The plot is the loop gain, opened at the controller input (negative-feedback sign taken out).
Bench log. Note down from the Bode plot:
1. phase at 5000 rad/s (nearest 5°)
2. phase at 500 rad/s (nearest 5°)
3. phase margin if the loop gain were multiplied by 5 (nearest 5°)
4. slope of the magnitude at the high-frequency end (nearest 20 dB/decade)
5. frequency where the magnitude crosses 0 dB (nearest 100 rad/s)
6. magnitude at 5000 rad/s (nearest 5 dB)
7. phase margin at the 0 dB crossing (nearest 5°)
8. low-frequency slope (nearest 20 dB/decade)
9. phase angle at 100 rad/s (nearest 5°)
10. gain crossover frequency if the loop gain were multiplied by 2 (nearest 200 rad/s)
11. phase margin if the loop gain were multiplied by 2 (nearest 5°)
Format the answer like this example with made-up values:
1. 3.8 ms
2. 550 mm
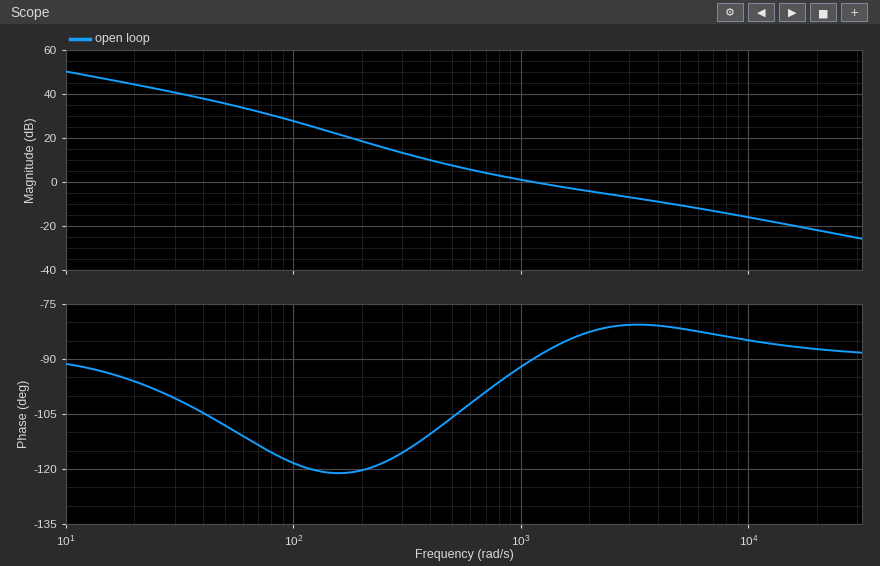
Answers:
1. -80°
2. -105°
3. 95°
4. -20 dB/decade
5. 1100 rad/s
6. -10 dB
7. 90°
8. -20 dB/decade
9. -120°
10. 2600 rad/s
11. 100°
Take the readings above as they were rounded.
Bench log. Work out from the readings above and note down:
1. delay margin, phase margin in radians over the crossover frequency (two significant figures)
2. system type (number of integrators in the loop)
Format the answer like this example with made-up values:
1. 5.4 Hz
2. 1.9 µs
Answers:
1. 0.0014 s
2. 1
